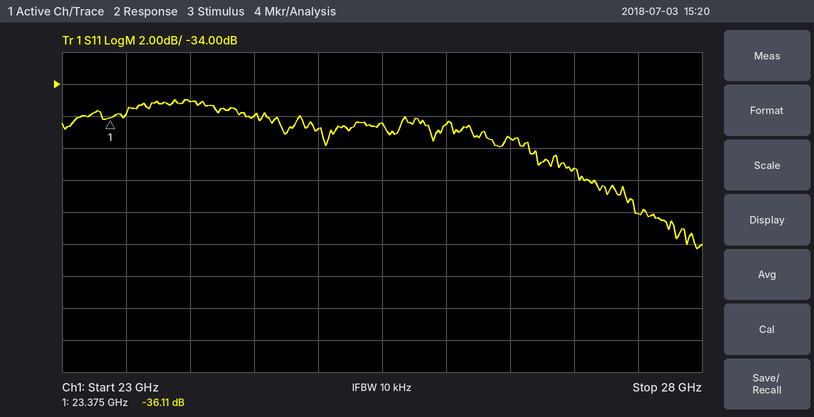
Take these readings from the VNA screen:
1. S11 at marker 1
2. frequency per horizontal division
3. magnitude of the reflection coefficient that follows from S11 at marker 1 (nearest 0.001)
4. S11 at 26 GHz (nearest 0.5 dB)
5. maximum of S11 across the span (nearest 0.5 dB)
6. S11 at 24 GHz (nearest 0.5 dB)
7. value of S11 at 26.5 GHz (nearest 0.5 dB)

-36.11 dB
500 MHz
0.016
-36.5 dB
-35.0 dB
-35.0 dB
-37.5 dB
